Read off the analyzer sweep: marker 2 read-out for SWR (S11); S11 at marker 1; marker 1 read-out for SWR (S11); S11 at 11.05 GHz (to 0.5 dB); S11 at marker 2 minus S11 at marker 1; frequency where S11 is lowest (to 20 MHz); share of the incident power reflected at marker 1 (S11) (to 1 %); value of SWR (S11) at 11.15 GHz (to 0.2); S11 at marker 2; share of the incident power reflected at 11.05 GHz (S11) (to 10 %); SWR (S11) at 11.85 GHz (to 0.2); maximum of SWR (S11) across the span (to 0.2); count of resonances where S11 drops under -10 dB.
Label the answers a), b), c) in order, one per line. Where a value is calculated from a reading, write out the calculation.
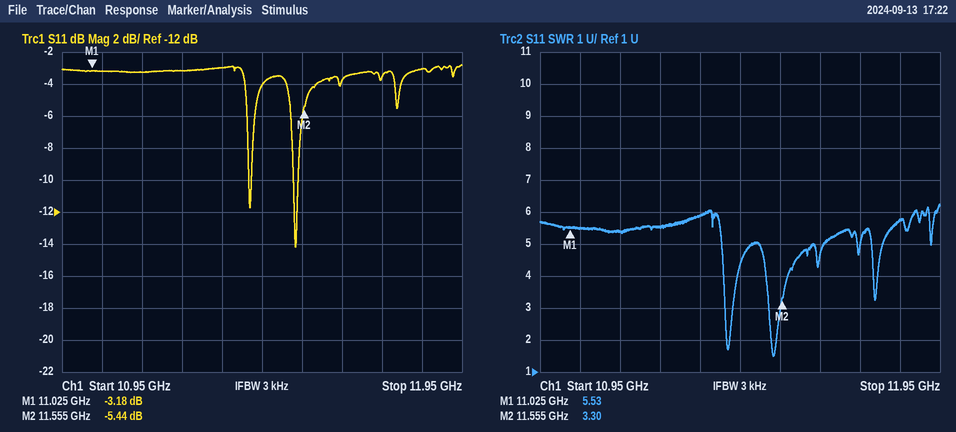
a) 3.30
b) -3.18 dB
c) 5.53
d) -3.0 dB
e) -5.44 − (-3.18) = -2.26 dB
f) 11.54 GHz
g) 10^(-3.18/10) ≈ 48 %
h) 5.4
i) -5.44 dB
j) 10^(-3/10) ≈ 50 %
k) 5.8
l) 6.2
m) 2
